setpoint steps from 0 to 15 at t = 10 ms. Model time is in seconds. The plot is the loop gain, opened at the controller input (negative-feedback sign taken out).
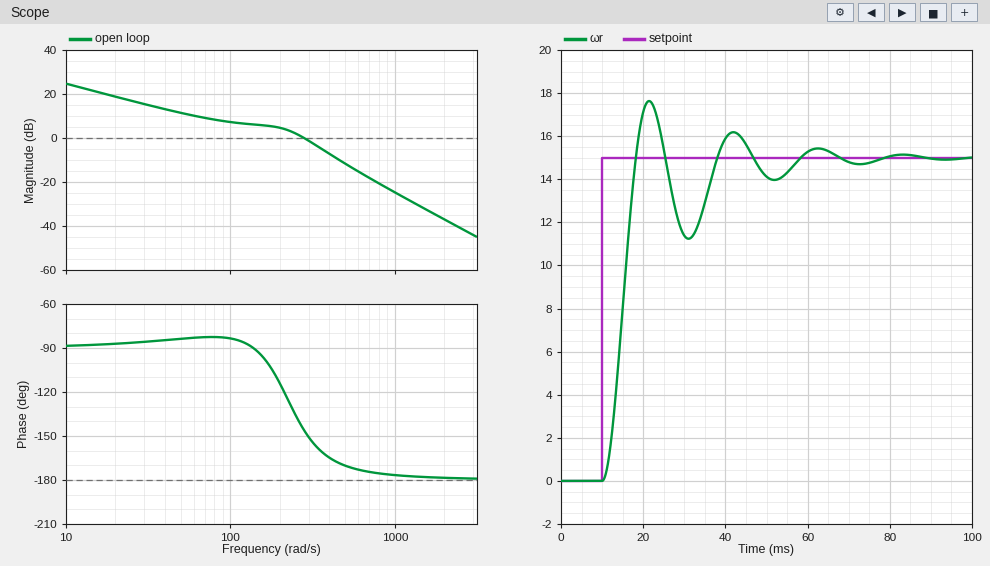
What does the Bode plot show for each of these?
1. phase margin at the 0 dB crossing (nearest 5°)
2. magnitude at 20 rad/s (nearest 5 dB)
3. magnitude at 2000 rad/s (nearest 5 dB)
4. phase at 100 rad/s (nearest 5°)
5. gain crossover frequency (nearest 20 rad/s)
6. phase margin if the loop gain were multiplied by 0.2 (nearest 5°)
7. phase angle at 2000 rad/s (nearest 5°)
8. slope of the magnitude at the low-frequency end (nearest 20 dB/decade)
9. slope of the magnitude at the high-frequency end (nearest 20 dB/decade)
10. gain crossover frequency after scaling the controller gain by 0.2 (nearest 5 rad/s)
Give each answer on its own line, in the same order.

35°
20 dB
-35 dB
-85°
280 rad/s
95°
-180°
-20 dB/decade
-40 dB/decade
35 rad/s
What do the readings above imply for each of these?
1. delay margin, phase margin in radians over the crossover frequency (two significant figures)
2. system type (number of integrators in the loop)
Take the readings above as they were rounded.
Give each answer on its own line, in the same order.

0.0022 s
1
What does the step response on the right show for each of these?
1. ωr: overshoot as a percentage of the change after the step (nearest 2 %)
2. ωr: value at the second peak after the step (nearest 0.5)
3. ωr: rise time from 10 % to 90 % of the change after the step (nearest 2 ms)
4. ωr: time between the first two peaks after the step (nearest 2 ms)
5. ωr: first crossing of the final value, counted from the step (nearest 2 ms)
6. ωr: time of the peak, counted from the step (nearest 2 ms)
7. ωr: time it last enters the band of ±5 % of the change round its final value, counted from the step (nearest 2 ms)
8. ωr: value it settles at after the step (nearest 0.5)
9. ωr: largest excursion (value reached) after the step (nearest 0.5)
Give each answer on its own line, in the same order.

18 %
16.0
6 ms
20 ms
8 ms
12 ms
44 ms
15.0
17.5
